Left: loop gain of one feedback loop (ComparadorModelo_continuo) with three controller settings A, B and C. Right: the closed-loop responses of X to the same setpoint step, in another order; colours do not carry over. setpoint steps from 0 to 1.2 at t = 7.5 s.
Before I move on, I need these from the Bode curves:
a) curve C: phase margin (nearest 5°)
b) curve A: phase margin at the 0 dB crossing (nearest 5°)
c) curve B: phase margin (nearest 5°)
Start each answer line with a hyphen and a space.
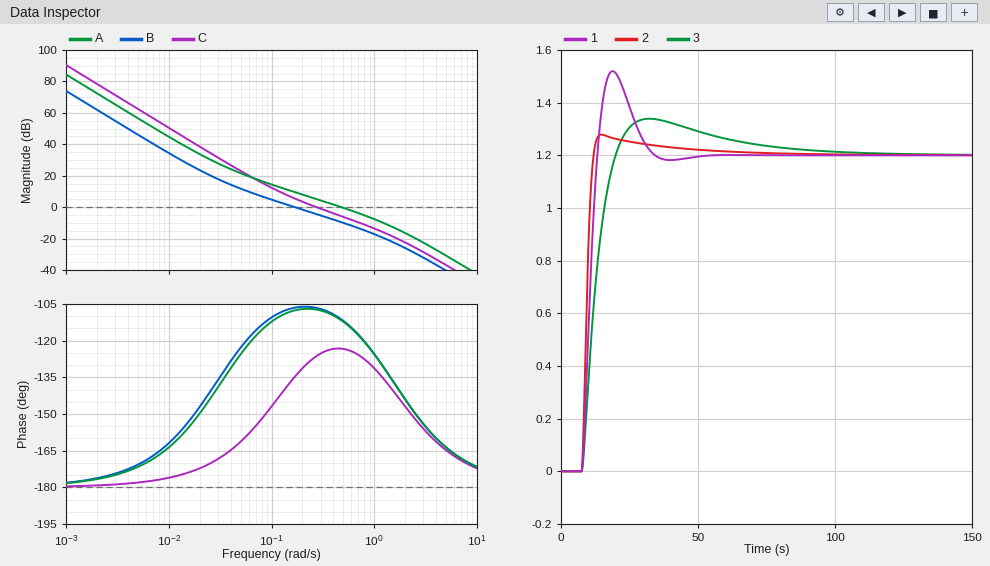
- 55°
- 70°
- 75°
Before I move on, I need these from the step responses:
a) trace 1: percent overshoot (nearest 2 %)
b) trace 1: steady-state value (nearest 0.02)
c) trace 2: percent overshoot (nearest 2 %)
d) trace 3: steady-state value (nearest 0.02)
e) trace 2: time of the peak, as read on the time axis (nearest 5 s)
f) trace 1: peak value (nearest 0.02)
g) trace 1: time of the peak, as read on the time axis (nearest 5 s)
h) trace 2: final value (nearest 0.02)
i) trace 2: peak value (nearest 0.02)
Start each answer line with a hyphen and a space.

- 26 %
- 1.20
- 6 %
- 1.20
- 15 s
- 1.52
- 20 s
- 1.20
- 1.28
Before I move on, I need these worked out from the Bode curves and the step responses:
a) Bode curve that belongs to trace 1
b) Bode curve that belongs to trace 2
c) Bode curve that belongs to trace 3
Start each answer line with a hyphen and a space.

- C
- A
- B
